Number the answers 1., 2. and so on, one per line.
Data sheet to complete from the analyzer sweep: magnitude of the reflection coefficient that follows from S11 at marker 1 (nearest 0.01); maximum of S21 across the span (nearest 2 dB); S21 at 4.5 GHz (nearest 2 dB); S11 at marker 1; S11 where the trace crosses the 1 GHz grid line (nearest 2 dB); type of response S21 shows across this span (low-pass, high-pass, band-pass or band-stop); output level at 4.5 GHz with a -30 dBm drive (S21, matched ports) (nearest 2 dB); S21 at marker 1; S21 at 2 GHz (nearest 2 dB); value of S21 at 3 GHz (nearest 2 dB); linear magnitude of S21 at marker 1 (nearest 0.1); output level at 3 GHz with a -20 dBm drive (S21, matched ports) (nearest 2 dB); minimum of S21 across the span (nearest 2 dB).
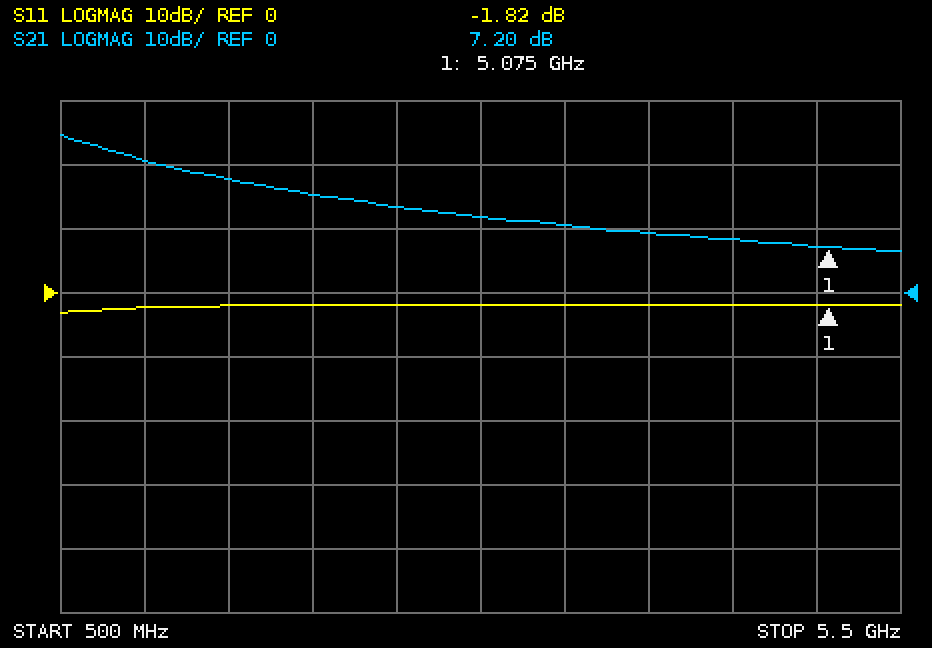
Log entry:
1. 0.81
2. 24 dB
3. 8 dB
4. -1.82 dB
5. -2 dB
6. low-pass
7. -22 dBm
8. 7.20 dB
9. 16 dB
10. 12 dB
11. 2.3
12. -8 dBm
13. 6 dB
